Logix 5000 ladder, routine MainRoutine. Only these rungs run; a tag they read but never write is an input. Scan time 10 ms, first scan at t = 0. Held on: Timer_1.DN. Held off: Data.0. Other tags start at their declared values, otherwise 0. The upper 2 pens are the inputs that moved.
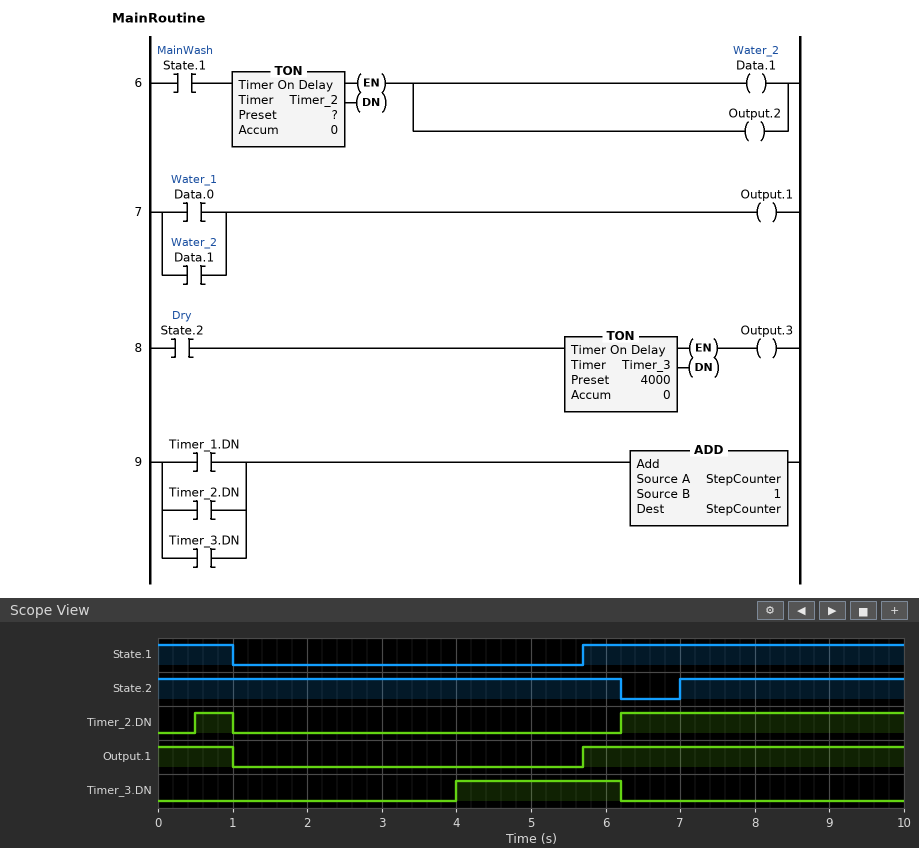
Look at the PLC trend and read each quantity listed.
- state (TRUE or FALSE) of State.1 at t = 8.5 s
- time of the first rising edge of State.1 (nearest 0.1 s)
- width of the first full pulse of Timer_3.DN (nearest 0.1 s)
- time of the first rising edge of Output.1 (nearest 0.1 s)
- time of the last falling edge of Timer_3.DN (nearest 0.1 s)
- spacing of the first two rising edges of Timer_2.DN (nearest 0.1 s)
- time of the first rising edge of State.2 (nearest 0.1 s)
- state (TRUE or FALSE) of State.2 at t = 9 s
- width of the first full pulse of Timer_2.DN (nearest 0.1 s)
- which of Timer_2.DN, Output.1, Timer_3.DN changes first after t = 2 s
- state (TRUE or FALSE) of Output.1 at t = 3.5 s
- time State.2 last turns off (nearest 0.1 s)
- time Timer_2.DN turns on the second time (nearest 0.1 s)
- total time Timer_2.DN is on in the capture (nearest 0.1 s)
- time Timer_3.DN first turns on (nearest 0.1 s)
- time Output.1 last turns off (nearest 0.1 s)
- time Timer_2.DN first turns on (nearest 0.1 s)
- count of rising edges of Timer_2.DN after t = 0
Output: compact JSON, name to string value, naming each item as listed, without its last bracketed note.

{"state (TRUE or FALSE) of State.1 at t = 8.5 s": "TRUE", "time of the first rising edge of State.1": "5.7 s", "width of the first full pulse of Timer_3.DN": "2.2 s", "time of the first rising edge of Output.1": "5.7 s", "time of the last falling edge of Timer_3.DN": "6.2 s", "spacing of the first two rising edges of Timer_2.DN": "5.7 s", "time of the first rising edge of State.2": "7.0 s", "state (TRUE or FALSE) of State.2 at t = 9 s": "TRUE", "width of the first full pulse of Timer_2.DN": "0.5 s", "which of Timer_2.DN, Output.1, Timer_3.DN changes first after t = 2 s": "Timer_3.DN", "state (TRUE or FALSE) of Output.1 at t = 3.5 s": "FALSE", "time State.2 last turns off": "6.2 s", "time Timer_2.DN turns on the second time": "6.2 s", "total time Timer_2.DN is on in the capture": "4.3 s", "time Timer_3.DN first turns on": "4.0 s", "time Output.1 last turns off": "1.0 s", "time Timer_2.DN first turns on": "0.5 s", "count of rising edges of Timer_2.DN after t = 0": "2"}
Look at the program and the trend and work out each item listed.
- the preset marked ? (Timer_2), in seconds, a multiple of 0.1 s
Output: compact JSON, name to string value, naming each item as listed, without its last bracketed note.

{"the preset marked ? (Timer_2), in seconds, a multiple of 0.1 s": "0.5 s"}
